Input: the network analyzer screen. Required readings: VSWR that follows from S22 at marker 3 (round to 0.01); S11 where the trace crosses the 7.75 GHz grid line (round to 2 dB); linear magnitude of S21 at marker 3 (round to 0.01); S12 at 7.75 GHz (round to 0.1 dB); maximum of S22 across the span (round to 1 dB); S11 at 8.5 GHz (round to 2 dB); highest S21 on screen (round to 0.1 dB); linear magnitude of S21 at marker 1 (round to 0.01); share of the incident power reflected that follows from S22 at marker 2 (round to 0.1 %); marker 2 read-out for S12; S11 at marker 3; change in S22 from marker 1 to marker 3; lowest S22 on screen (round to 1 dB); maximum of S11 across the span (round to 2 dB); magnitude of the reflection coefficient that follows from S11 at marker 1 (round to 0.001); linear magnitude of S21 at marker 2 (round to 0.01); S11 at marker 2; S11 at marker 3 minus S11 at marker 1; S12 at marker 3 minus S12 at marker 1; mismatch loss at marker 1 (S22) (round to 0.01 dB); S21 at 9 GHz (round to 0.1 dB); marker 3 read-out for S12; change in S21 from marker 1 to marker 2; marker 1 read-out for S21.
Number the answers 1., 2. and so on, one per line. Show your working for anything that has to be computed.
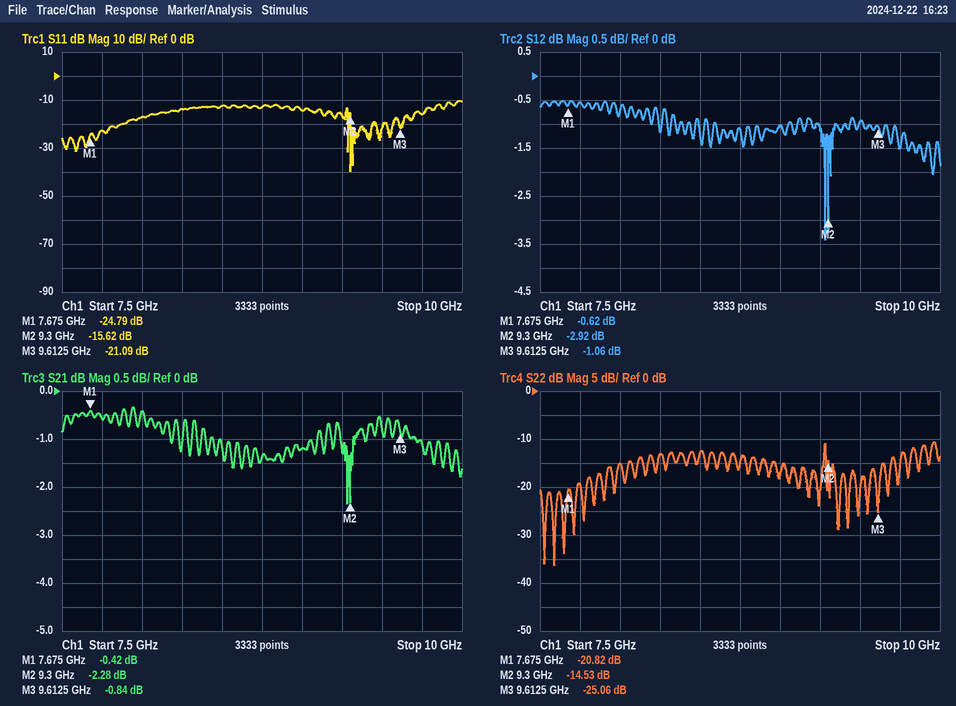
1. (1 + 0.0558)/(1 − 0.0558) ≈ 1.12
2. -22 dB
3. 10^(-0.84/20) ≈ 0.91
4. -0.5 dB
5. -11 dB
6. -12 dB
7. -0.3 dB
8. 10^(-0.42/20) ≈ 0.95
9. 10^(-14.53/10) ≈ 3.5 %
10. -2.92 dB
11. -21.09 dB
12. -25.06 − (-20.82) = -4.24 dB
13. -36 dB
14. -10 dB
15. 10^(-24.79/20) ≈ 0.058
16. 10^(-2.28/20) ≈ 0.77
17. -15.62 dB
18. -21.09 − (-24.79) = 3.70 dB
19. -1.06 − (-0.62) = -0.44 dB
20. −10 log10(1 − 10^(-20.82/10)) ≈ 0.04 dB
21. -1.2 dB
22. -1.06 dB
23. -2.28 − (-0.42) = -1.86 dB
24. -0.42 dB
